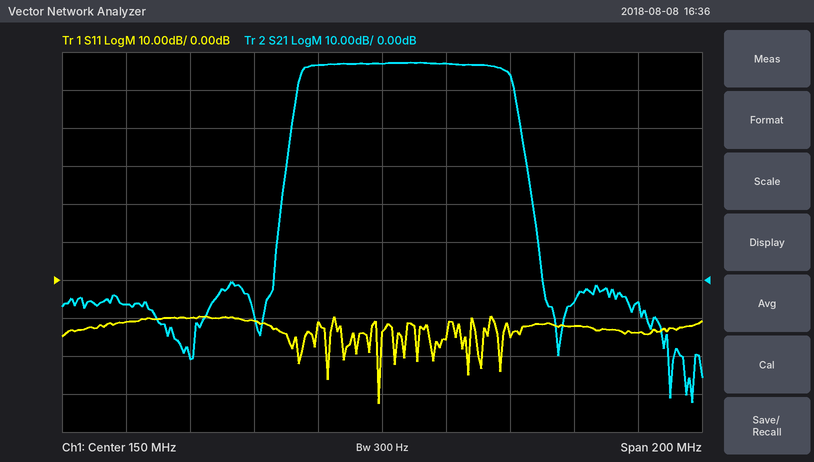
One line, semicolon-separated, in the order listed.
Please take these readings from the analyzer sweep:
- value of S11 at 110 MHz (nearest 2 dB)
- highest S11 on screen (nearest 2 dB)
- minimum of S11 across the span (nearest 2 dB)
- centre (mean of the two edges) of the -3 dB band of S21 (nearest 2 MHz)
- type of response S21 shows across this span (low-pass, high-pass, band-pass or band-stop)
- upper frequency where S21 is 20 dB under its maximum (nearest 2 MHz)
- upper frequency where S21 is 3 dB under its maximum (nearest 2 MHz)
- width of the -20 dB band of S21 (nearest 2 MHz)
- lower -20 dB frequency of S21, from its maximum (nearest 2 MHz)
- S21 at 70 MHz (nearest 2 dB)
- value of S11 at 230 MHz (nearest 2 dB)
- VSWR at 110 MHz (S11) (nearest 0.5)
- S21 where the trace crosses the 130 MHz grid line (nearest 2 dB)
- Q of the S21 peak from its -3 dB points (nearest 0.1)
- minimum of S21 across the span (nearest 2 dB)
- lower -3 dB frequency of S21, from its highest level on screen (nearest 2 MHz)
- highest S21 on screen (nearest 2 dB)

-10 dB; -10 dB; -32 dB; 158 MHz; band-pass; 194 MHz; 190 MHz; 72 MHz; 122 MHz; -6 dB; -14 dB; 2.0; 56 dB; 2.4; -32 dB; 124 MHz; 58 dB
